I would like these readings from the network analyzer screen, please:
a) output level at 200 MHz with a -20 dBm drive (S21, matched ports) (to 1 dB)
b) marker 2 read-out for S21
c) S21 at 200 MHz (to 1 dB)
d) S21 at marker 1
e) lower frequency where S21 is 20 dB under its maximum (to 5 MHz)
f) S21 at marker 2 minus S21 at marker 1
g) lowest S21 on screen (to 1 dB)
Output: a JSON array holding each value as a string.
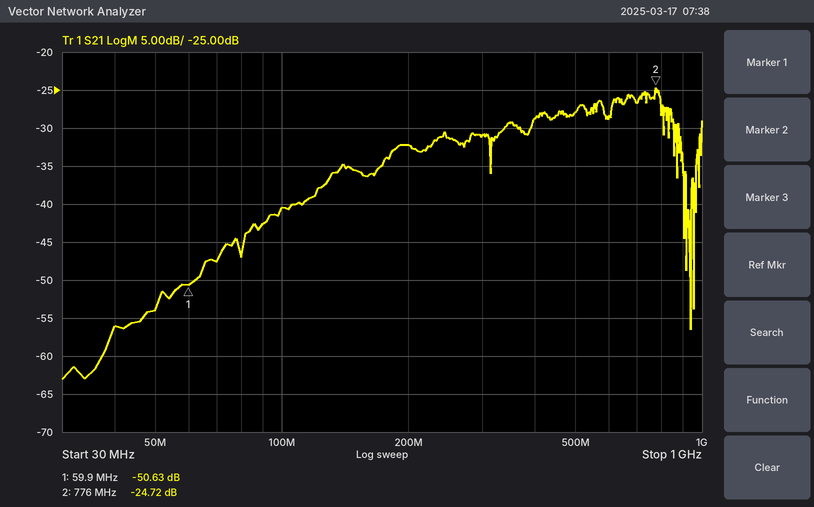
["-52 dBm", "-24.72 dB", "-32 dB", "-50.63 dB", "80 MHz", "25.91 dB", "-63 dB"]
